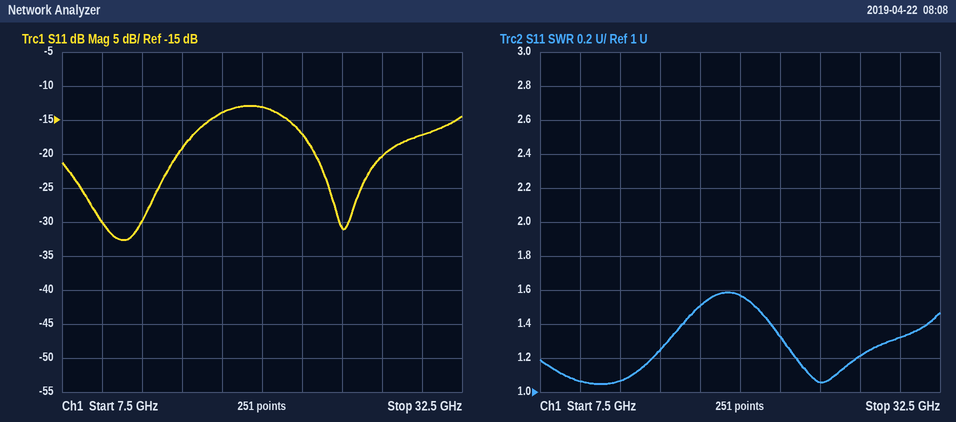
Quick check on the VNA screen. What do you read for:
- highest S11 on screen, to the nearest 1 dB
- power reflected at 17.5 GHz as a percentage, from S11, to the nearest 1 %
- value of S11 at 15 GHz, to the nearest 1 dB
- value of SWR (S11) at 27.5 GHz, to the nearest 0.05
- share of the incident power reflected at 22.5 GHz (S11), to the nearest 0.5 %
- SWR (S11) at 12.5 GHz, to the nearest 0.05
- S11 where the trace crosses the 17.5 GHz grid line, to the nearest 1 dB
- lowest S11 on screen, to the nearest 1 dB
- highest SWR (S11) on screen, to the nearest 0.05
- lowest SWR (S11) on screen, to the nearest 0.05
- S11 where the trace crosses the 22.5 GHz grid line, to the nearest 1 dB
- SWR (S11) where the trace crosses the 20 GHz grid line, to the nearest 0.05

-13 dB
4 %
-19 dB
1.20
2.0 %
1.05
-14 dB
-33 dB
1.60
1.05
-17 dB
1.55
